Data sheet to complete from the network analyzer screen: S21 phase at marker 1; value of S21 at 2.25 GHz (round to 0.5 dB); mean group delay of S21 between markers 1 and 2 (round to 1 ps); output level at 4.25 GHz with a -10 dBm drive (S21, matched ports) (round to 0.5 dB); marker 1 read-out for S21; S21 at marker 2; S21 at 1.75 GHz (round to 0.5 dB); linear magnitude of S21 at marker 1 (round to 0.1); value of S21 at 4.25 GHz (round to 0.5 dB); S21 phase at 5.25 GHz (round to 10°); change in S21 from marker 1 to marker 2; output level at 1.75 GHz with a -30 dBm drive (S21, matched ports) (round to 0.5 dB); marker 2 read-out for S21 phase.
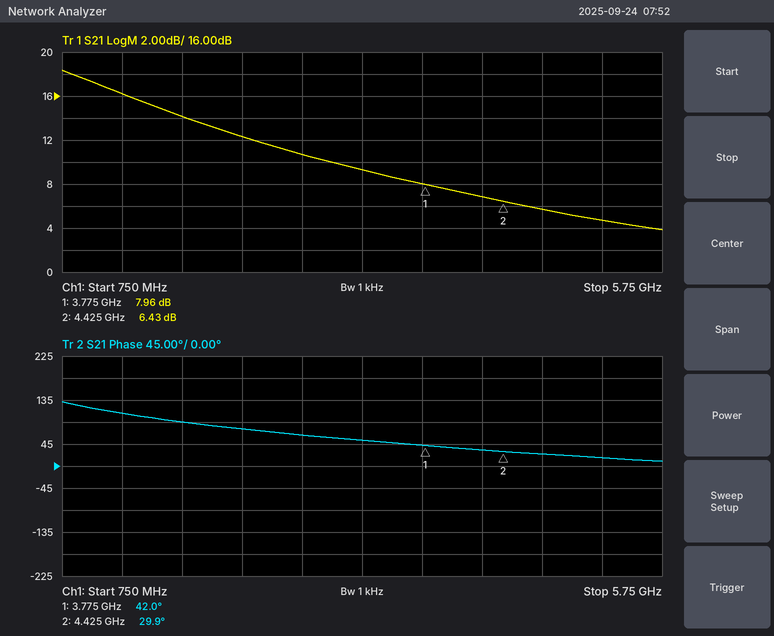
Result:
42.0°
12.5 dB
52 ps
-3.0 dBm
7.96 dB
6.43 dB
14.0 dB
2.5
7.0 dB
20°
-1.53 dB
-16.0 dBm
29.9°
